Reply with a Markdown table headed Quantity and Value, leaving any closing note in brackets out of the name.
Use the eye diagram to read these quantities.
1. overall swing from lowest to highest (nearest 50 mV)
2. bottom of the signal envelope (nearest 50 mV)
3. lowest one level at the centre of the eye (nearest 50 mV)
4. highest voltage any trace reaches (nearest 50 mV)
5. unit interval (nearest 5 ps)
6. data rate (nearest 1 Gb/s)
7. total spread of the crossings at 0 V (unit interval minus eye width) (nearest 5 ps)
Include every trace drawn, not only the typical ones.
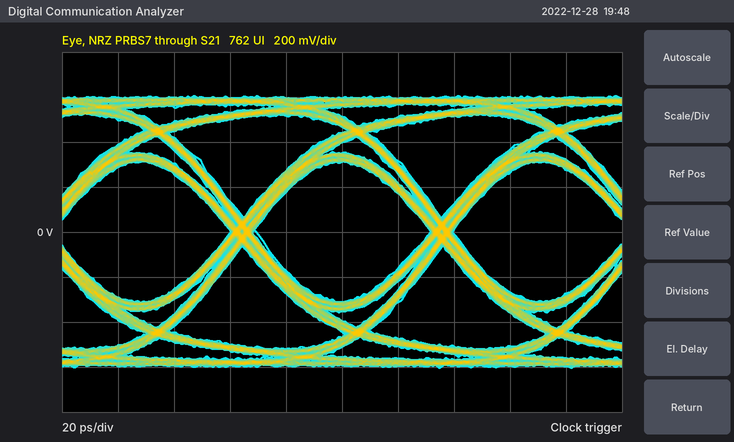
| Quantity | Value |
|---|---|
| overall swing from lowest to highest | 1.20 V |
| bottom of the signal envelope | -600 mV |
| lowest one level at the centre of the eye | 300 mV |
| highest voltage any trace reaches | 600 mV |
| unit interval | 70 ps |
| data rate | 14 Gb/s |
| total spread of the crossings at 0 V (unit interval minus eye width) | 10 ps |
